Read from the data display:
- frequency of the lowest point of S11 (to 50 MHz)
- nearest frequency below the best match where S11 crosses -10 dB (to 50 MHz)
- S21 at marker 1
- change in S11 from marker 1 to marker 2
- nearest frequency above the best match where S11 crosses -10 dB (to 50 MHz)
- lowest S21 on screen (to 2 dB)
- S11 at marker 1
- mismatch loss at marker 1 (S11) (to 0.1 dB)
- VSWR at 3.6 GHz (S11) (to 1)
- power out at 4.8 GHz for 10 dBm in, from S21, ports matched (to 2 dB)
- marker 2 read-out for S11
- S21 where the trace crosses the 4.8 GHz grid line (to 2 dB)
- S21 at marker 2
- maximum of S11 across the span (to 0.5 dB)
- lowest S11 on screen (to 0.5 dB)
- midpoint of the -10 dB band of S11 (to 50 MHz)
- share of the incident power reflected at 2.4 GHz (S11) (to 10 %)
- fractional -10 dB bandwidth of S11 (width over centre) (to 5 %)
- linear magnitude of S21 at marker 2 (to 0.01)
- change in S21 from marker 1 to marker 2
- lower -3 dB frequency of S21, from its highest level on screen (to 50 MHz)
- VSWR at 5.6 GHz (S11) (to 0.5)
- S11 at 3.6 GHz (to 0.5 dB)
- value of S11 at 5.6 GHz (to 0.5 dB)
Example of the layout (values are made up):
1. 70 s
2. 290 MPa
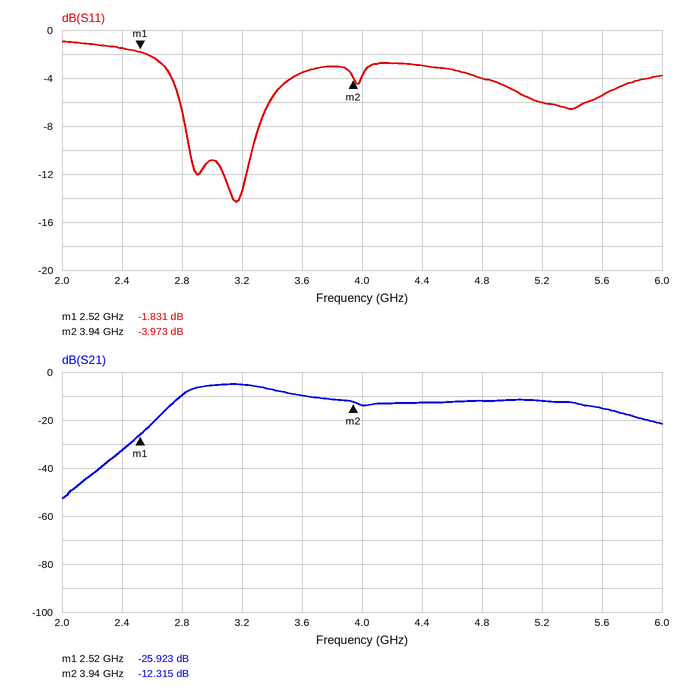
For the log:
1. 3.15 GHz
2. 2.85 GHz
3. -25.923 dB
4. -2.142 dB
5. 3.25 GHz
6. -52 dB
7. -1.831 dB
8. 4.6 dB
9. 5
10. -2 dBm
11. -3.973 dB
12. -12 dB
13. -12.315 dB
14. -1.0 dB
15. -14.5 dB
16. 3.05 GHz
17. 70 %
18. 15 %
19. 0.24
20. 13.608 dB
21. 2.85 GHz
22. 3.5
23. -3.5 dB
24. -5.5 dB
